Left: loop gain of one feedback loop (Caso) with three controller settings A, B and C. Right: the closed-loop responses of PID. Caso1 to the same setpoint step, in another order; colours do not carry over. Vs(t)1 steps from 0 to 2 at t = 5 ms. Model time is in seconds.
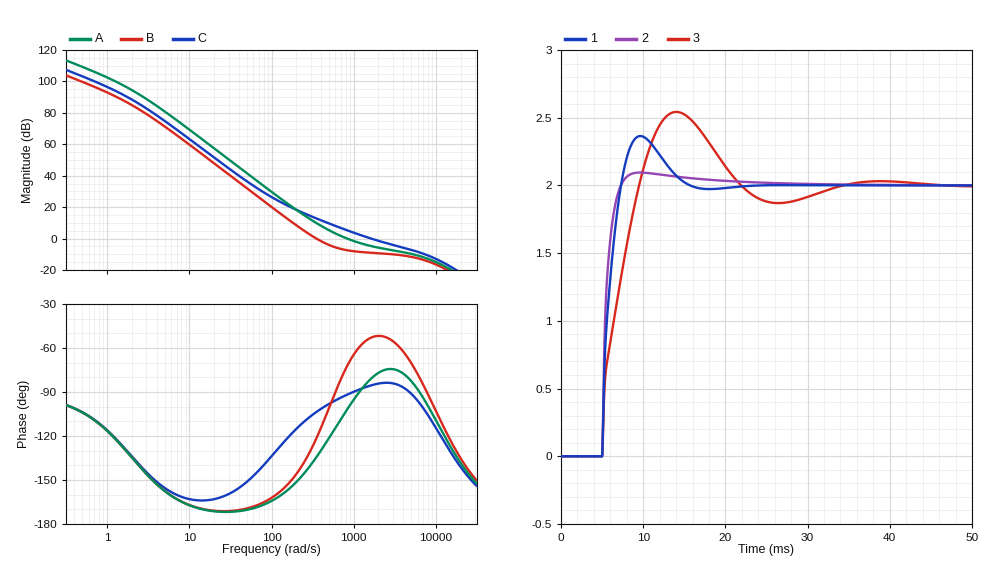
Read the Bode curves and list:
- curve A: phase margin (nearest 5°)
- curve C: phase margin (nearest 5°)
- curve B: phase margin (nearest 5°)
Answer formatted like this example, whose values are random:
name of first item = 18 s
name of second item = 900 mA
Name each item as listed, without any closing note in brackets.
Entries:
curve A: phase margin = 80°
curve C: phase margin = 95°
curve B: phase margin = 60°
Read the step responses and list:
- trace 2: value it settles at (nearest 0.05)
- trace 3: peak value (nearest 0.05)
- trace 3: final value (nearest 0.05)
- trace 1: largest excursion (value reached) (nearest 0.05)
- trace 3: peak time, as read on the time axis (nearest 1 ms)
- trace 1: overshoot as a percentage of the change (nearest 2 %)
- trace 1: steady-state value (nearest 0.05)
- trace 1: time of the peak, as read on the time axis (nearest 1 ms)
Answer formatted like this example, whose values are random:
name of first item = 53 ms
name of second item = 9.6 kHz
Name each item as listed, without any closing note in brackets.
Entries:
trace 2: value it settles at = 2.00
trace 3: peak value = 2.55
trace 3: final value = 2.00
trace 1: largest excursion (value reached) = 2.35
trace 3: peak time, as read on the time axis = 14 ms
trace 1: overshoot as a percentage of the change = 18 %
trace 1: steady-state value = 2.00
trace 1: time of the peak, as read on the time axis = 10 ms
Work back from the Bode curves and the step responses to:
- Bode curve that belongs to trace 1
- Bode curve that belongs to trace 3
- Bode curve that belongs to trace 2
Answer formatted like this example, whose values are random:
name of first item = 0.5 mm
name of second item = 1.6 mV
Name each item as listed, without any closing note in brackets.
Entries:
Bode curve that belongs to trace 1 = A
Bode curve that belongs to trace 3 = B
Bode curve that belongs to trace 2 = C
